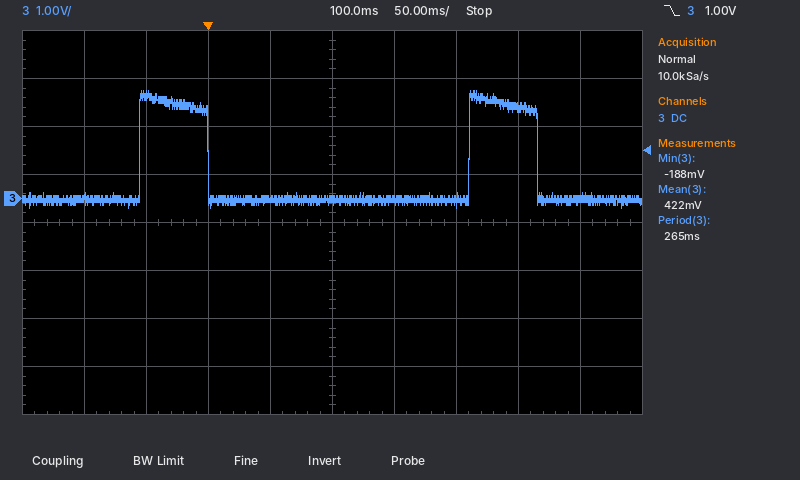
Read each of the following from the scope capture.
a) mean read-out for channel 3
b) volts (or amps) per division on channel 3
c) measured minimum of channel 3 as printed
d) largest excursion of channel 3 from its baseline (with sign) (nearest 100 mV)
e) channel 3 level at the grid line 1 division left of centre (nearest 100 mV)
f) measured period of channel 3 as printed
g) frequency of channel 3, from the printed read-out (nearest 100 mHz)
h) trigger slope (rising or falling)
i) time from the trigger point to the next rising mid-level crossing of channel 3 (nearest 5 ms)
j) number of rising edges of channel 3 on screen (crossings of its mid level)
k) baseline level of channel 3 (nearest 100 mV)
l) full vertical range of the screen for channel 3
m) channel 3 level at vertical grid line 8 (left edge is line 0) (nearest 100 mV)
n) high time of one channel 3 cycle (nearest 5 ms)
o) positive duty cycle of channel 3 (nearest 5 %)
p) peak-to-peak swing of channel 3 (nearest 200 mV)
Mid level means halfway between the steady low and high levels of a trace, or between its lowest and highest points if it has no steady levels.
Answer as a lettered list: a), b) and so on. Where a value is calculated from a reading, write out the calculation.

a) 422 mV
b) 1 V
c) -188 mV
d) +2.3 V
e) 0.0 V
f) 265 ms
g) 1 / 265 ms ≈ 3.8 Hz
h) falling
i) 210 ms
j) 2
k) 0.0 V
l) 8 V
m) 1.9 V
n) 55 ms
o) 20 %
p) 2.4 V
